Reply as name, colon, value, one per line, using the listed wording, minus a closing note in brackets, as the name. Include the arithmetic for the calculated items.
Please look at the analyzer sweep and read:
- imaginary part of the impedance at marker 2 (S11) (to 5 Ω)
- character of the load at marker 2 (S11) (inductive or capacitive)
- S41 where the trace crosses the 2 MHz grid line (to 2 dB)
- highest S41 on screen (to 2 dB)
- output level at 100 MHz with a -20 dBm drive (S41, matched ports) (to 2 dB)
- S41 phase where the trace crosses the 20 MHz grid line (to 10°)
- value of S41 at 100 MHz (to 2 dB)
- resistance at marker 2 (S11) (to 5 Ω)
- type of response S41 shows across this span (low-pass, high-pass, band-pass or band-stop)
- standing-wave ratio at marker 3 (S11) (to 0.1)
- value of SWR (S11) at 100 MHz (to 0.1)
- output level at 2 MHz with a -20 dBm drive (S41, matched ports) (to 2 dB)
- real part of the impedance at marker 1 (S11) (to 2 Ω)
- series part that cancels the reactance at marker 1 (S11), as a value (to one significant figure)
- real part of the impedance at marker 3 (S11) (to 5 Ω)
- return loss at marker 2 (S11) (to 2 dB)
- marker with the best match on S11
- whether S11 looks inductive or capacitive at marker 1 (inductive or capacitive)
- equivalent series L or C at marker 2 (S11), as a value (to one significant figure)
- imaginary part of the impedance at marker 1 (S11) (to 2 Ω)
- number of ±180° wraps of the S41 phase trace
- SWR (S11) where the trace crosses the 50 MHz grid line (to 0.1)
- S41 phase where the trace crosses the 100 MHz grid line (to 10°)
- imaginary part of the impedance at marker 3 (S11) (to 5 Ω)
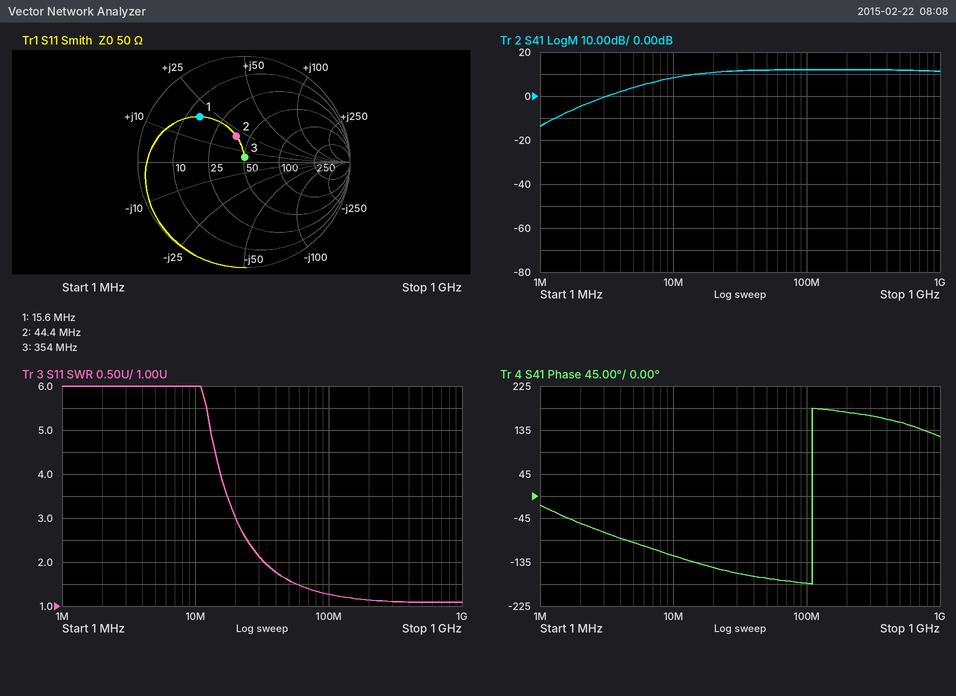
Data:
imaginary part of the impedance at marker 2 (S11): +20 Ω
character of the load at marker 2 (S11): inductive
S41 where the trace crosses the 2 MHz grid line: -4 dB
highest S41 on screen: 12 dB
output level at 100 MHz with a -20 dBm drive (S41, matched ports): -20 dBm + (12 dB) = -8 dBm
S41 phase where the trace crosses the 20 MHz grid line: -150°
value of S41 at 100 MHz: 12 dB
resistance at marker 2 (S11): 40 Ω
type of response S41 shows across this span: high-pass
standing-wave ratio at marker 3 (S11): 1.1
value of SWR (S11) at 100 MHz: 1.3
output level at 2 MHz with a -20 dBm drive (S41, matched ports): -20 dBm + (-4 dB) = -24 dBm
real part of the impedance at marker 1 (S11): 14 Ω
series part that cancels the reactance at marker 1 (S11), as a value: C = 1/(2π × 15.6 MHz × 20 Ω) ≈ 510 pF, so 500 pF to one significant figure
real part of the impedance at marker 3 (S11): 50 Ω
return loss at marker 2 (S11): 12 dB
marker with the best match on S11: marker 3
whether S11 looks inductive or capacitive at marker 1: inductive
equivalent series L or C at marker 2 (S11), as a value: L = 20 Ω/(2π × 44.4 MHz) ≈ 71.7 nH, so 70 nH to one significant figure
imaginary part of the impedance at marker 1 (S11): +20 Ω
number of ±180° wraps of the S41 phase trace: 1
SWR (S11) where the trace crosses the 50 MHz grid line: 1.6
S41 phase where the trace crosses the 100 MHz grid line: -180°
imaginary part of the impedance at marker 3 (S11): +5 Ω
